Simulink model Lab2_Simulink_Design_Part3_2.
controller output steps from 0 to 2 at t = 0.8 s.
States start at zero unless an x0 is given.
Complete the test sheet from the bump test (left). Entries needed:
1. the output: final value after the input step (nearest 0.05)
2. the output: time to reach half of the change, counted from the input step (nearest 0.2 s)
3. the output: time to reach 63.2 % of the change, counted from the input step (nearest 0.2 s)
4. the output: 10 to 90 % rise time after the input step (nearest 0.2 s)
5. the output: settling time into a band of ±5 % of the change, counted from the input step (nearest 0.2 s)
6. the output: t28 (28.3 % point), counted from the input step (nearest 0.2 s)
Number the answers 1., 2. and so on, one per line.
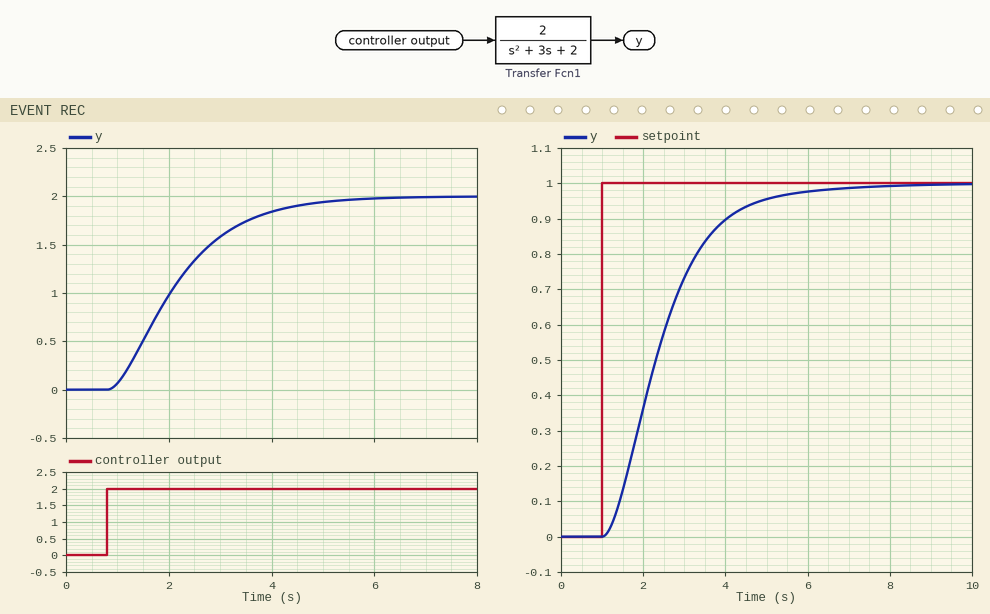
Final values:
1. 2.00
2. 1.2 s
3. 1.6 s
4. 2.6 s
5. 3.6 s
6. 0.8 s
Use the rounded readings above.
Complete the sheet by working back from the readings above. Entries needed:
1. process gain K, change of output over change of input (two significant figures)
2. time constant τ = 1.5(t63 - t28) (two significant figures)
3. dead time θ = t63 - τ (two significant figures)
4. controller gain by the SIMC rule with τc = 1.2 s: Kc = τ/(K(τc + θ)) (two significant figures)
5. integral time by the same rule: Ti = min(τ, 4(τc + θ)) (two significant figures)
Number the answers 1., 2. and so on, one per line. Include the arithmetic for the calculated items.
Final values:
1. (2 - 0) / 2 = 1.0
2. 1.5 × (1.6 - 0.8) = 1.2 s
3. 1.6 - 1.2 = 0.40 s
4. 1.2 / (1 × (1.2 + 0.4)) = 0.75
5. min(1.2, 4 × (1.2 + 0.4)) = 1.2 s
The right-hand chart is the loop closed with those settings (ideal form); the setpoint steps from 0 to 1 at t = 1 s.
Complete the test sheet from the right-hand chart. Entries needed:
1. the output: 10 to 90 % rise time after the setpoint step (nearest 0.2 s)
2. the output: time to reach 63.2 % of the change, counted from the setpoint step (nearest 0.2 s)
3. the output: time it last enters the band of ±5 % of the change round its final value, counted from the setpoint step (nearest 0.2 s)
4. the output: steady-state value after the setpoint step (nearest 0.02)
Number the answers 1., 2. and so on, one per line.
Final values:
1. 2.6 s
2. 1.6 s
3. 3.8 s
4. 1.00
